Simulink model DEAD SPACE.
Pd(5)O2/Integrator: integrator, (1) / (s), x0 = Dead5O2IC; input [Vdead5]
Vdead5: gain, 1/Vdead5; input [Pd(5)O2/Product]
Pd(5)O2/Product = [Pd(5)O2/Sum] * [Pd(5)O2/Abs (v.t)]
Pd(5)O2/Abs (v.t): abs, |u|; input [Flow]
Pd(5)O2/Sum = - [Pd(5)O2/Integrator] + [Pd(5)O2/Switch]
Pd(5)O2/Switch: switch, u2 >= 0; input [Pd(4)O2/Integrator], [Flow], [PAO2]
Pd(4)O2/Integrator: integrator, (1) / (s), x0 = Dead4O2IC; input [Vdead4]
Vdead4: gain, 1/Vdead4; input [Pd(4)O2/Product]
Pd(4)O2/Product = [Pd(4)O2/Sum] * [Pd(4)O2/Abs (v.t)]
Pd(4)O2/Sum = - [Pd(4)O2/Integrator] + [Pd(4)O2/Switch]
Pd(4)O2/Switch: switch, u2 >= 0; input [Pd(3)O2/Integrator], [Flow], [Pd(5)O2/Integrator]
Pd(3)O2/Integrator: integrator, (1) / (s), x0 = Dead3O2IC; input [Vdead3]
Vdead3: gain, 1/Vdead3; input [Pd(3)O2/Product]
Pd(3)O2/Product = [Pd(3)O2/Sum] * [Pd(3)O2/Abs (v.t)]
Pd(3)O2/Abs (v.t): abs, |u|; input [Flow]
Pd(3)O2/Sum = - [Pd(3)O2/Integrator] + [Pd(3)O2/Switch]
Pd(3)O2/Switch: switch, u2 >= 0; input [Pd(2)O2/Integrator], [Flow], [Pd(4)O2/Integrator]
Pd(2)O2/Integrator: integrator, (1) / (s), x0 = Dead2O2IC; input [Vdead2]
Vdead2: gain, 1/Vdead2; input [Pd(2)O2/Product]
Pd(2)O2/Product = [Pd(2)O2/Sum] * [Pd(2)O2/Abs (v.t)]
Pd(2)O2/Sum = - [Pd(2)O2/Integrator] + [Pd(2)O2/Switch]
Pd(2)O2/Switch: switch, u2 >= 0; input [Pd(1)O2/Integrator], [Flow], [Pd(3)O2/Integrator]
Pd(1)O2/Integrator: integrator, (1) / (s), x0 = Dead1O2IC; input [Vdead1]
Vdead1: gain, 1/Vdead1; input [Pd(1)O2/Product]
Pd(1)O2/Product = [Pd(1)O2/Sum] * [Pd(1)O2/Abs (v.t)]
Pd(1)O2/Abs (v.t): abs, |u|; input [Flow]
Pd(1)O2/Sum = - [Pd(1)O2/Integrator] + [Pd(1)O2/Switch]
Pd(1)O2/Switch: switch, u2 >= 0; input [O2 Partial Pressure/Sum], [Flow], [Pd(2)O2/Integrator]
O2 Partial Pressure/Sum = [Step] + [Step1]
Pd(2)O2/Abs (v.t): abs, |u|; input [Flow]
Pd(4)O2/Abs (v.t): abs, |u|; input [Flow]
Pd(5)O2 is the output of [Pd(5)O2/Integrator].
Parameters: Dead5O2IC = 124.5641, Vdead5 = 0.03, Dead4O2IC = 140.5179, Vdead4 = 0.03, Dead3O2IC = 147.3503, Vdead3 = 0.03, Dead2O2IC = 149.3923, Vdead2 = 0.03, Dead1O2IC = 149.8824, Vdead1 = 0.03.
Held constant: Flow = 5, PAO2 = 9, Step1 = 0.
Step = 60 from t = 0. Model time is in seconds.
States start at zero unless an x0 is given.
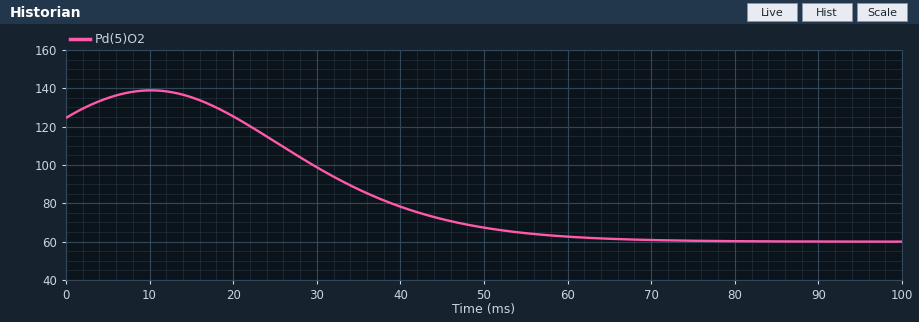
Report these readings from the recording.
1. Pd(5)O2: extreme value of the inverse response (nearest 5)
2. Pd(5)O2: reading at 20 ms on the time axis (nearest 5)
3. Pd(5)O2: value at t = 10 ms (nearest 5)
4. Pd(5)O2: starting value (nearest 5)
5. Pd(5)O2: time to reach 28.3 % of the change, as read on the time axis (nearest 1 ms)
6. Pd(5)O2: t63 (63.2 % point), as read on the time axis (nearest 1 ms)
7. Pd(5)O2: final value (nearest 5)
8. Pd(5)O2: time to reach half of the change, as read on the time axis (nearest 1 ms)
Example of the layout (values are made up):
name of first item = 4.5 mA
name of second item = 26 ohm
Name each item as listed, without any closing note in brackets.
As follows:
Pd(5)O2: extreme value of the inverse response = 140
Pd(5)O2: reading at 20 ms on the time axis = 125
Pd(5)O2: value at t = 10 ms = 140
Pd(5)O2: starting value = 125
Pd(5)O2: time to reach 28.3 % of the change, as read on the time axis = 27 ms
Pd(5)O2: t63 (63.2 % point), as read on the time axis = 37 ms
Pd(5)O2: final value = 60
Pd(5)O2: time to reach half of the change, as read on the time axis = 33 ms
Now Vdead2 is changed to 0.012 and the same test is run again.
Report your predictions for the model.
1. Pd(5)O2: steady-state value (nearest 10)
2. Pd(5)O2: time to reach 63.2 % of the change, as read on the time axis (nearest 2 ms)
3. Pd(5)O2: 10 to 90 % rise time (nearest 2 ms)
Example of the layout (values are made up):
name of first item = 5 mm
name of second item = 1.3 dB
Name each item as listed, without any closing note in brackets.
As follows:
Pd(5)O2: steady-state value = 60
Pd(5)O2: time to reach 63.2 % of the change, as read on the time axis = 32 ms
Pd(5)O2: 10 to 90 % rise time = 26 ms
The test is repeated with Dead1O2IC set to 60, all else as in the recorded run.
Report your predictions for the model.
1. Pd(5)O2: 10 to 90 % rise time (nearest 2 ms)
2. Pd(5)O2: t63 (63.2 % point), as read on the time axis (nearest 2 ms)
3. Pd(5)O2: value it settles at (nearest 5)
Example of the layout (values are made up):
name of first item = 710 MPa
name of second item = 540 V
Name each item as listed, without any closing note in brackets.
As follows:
Pd(5)O2: 10 to 90 % rise time = 26 ms
Pd(5)O2: t63 (63.2 % point), as read on the time axis = 30 ms
Pd(5)O2: value it settles at = 60
